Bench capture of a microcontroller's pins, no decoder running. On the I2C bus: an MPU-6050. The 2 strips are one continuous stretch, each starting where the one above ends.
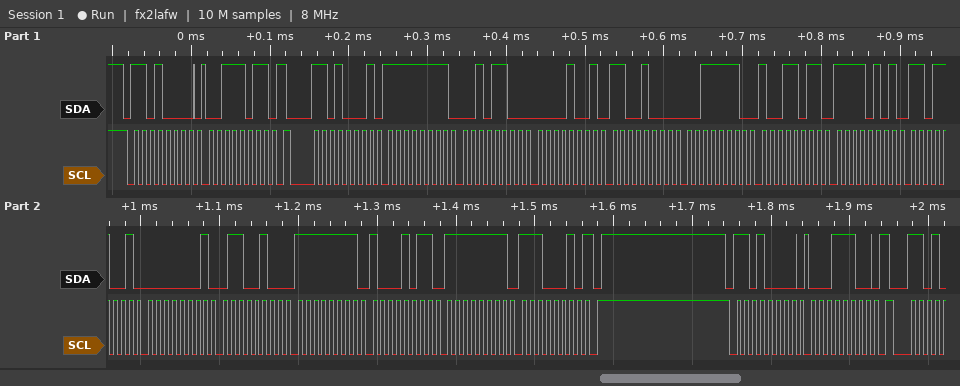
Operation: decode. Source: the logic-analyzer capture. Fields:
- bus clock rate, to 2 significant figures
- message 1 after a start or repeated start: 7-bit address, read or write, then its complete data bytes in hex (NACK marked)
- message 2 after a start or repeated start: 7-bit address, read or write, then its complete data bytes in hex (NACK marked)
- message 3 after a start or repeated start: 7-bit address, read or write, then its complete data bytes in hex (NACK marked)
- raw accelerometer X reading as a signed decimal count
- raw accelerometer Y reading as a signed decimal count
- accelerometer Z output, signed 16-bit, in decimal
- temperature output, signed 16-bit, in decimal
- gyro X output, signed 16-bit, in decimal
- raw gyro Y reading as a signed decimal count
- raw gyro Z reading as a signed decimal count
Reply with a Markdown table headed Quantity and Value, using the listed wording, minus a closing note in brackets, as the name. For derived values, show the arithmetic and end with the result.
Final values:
| Quantity | Value |
|---|---|
| bus clock rate, to 2 significant figures | 100 kHz |
| message 1 after a start or repeated start: 7-bit address, read or write, then its complete data bytes in hex | 0x68 write: 3B |
| message 2 after a start or repeated start: 7-bit address, read or write, then its complete data bytes in hex | 0x68 read: FF 2C 09 C8 3E 9B F5 D9 01 64 FF 8B FF E2 NACK |
| message 3 after a start or repeated start: 7-bit address, read or write, then its complete data bytes in hex | 0x68 write: 1C |
| raw accelerometer X reading as a signed decimal count | 0xFF2C = -212 |
| raw accelerometer Y reading as a signed decimal count | 0x09C8 = 2504 |
| accelerometer Z output, signed 16-bit, in decimal | 0x3E9B = 16027 |
| temperature output, signed 16-bit, in decimal | 0xF5D9 = -2599 |
| gyro X output, signed 16-bit, in decimal | 0x0164 = 356 |
| raw gyro Y reading as a signed decimal count | 0xFF8B = -117 |
| raw gyro Z reading as a signed decimal count | 0xFFE2 = -30 |
